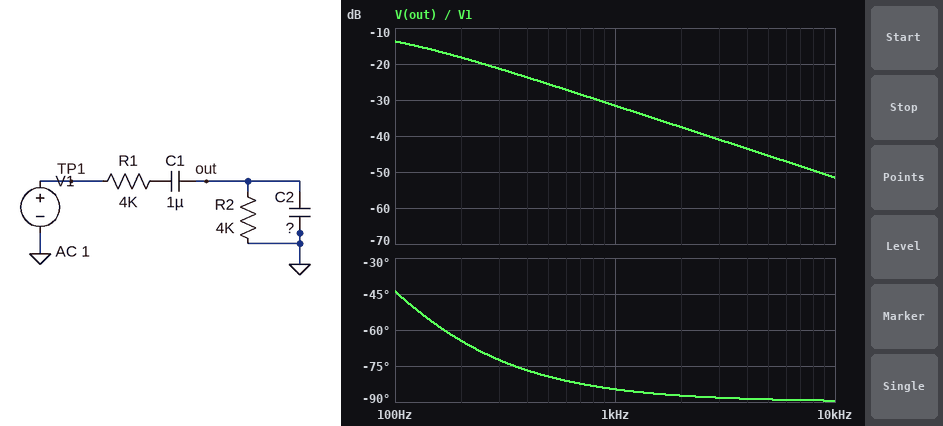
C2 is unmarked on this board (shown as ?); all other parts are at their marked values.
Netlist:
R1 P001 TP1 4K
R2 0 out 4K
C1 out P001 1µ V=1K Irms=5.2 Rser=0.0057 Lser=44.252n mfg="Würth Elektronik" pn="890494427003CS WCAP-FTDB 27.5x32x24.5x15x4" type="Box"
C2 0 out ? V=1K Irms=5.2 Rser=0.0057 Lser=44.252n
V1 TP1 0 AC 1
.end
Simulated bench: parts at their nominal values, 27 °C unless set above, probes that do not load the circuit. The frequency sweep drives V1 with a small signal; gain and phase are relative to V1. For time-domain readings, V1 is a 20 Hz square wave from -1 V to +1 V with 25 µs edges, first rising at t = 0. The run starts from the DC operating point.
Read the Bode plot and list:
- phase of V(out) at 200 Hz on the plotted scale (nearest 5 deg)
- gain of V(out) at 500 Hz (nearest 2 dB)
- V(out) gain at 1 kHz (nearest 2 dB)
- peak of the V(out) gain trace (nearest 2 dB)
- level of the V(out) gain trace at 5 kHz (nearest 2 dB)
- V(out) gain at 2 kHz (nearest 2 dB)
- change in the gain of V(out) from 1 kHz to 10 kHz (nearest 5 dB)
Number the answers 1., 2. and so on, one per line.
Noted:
1. -65 deg
2. -26 dB
3. -32 dB
4. -14 dB
5. -46 dB
6. -38 dB
7. -20 dB
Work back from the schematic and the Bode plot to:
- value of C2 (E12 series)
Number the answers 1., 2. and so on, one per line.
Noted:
1. 1.5 µF
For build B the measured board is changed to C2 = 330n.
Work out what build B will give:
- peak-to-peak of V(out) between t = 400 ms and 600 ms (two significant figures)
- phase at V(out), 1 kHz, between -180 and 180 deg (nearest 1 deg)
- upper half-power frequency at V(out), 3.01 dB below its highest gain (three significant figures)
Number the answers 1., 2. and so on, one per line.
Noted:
1. 1.4 V
2. -74 deg
3. 297 Hz
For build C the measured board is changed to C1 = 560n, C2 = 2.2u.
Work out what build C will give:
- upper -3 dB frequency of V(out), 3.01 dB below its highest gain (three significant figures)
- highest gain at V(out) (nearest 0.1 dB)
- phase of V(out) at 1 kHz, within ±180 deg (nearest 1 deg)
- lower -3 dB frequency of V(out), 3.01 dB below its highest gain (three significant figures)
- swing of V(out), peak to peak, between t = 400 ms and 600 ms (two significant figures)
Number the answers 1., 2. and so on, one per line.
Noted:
1. 118 Hz
2. -15.5 dB
3. -84 deg
4. 10.9 Hz
5. 490 mV
